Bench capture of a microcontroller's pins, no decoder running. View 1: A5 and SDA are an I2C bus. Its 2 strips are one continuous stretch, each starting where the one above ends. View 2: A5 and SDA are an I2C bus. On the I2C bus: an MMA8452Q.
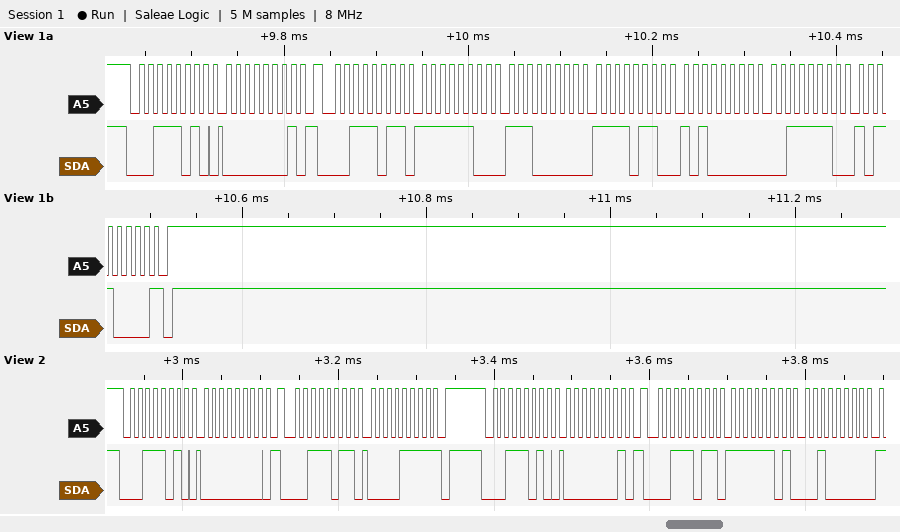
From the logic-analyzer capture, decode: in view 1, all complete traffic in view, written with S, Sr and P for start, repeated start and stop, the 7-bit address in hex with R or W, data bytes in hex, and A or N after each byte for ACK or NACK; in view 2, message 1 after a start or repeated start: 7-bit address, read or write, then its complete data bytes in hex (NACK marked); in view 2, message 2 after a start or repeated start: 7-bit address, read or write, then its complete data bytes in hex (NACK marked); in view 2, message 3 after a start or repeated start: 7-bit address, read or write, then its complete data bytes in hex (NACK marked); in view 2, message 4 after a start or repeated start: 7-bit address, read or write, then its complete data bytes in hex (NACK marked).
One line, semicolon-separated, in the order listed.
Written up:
S 1DW A 01 A Sr 1DR A FC A E0 A F6 A A0 A 3E A B0 N P; 0x1D write: 00; 0x1D read: 0F NACK; 0x1D write: 01; 0x1D read: FD 20
